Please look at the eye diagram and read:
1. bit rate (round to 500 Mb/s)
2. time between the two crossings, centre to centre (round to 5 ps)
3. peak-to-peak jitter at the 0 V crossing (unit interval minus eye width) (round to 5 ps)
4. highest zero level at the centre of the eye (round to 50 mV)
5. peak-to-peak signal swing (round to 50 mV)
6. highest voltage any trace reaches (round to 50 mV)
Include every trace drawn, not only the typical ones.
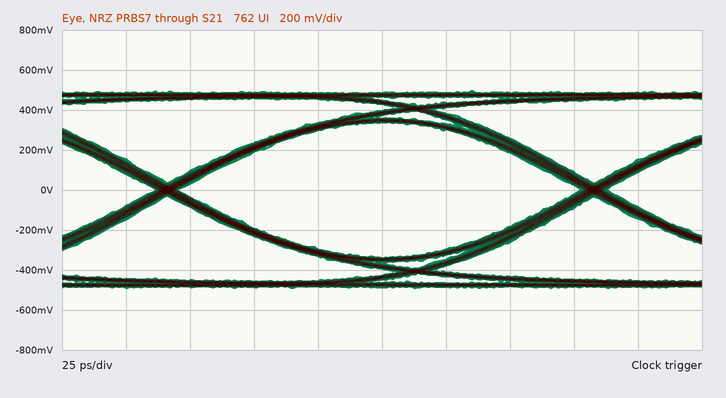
6.0 Gb/s
165 ps
10 ps
-350 mV
1.00 V
500 mV
